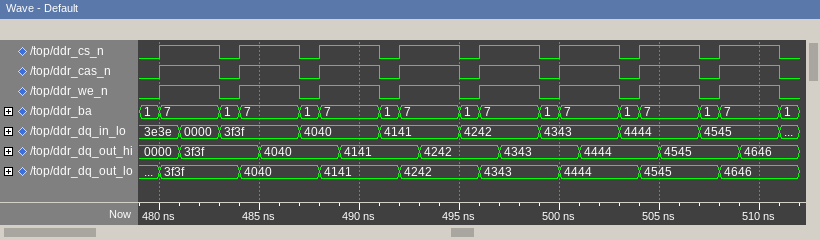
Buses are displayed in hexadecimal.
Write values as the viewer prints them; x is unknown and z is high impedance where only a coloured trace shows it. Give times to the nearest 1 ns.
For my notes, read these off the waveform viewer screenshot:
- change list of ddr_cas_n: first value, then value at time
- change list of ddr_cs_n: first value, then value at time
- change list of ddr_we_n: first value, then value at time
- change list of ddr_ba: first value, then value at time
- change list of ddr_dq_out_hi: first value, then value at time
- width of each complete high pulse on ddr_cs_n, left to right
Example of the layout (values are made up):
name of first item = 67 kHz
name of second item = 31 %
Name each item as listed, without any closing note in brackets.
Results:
change list of ddr_cas_n: first value, then value at time = 0, 1 at 480 ns, 0 at 483 ns, 1 at 484 ns, 0 at 487 ns, 1 at 488 ns, 0 at 491 ns, 1 at 492 ns, 0 at 495 ns, 1 at 496 ns, 0 at 499 ns, 1 at 500 ns, 0 at 503 ns, 1 at 504 ns, 0 at 507 ns, 1 at 508 ns, 0 at 511 ns
change list of ddr_cs_n: first value, then value at time = 0, 1 at 480 ns, 0 at 483 ns, 1 at 484 ns, 0 at 487 ns, 1 at 488 ns, 0 at 491 ns, 1 at 492 ns, 0 at 495 ns, 1 at 496 ns, 0 at 499 ns, 1 at 500 ns, 0 at 503 ns, 1 at 504 ns, 0 at 507 ns, 1 at 508 ns, 0 at 511 ns
change list of ddr_we_n: first value, then value at time = 0, 1 at 480 ns, 0 at 483 ns, 1 at 484 ns, 0 at 487 ns, 1 at 488 ns, 0 at 491 ns, 1 at 492 ns, 0 at 495 ns, 1 at 496 ns, 0 at 499 ns, 1 at 500 ns, 0 at 503 ns, 1 at 504 ns, 0 at 507 ns, 1 at 508 ns, 0 at 511 ns
change list of ddr_ba: first value, then value at time = 1, 7 at 480 ns, 1 at 483 ns, 7 at 484 ns, 1 at 487 ns, 7 at 488 ns, 1 at 491 ns, 7 at 492 ns, 1 at 495 ns, 7 at 496 ns, 1 at 499 ns, 7 at 500 ns, 1 at 503 ns, 7 at 504 ns, 1 at 507 ns, 7 at 508 ns, 1 at 511 ns
change list of ddr_dq_out_hi: first value, then value at time = 0000, 3f3f at 481 ns, 4040 at 485 ns, 4141 at 489 ns, 4242 at 493 ns, 4343 at 497 ns, 4444 at 501 ns, 4545 at 505 ns, 4646 at 509 ns
width of each complete high pulse on ddr_cs_n, left to right = 3 ns, 3 ns, 3 ns, 3 ns, 3 ns, 3 ns, 3 ns, 3 ns
